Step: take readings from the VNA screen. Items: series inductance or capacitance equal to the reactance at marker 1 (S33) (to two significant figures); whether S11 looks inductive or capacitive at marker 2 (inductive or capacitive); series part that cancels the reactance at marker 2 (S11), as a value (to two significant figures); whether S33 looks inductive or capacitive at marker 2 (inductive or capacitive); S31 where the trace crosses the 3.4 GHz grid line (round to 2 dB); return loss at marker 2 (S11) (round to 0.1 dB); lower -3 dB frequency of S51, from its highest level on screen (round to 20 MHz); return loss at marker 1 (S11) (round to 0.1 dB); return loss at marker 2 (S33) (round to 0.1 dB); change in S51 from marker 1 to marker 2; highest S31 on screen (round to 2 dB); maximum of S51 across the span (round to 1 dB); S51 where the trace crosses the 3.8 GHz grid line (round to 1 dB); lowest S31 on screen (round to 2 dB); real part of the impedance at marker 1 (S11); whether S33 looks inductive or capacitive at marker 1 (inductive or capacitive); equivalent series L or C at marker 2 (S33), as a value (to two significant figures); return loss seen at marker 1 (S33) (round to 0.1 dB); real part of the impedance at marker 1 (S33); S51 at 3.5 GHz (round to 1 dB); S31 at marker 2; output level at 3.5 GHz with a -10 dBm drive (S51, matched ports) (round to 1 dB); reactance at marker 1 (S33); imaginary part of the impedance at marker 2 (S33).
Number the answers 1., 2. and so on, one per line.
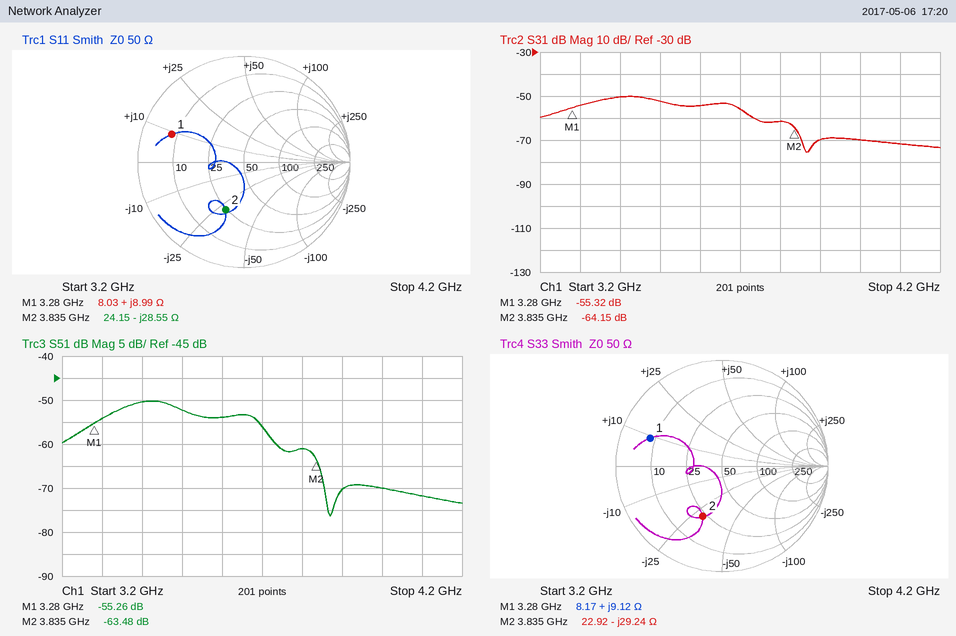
1. 440 pH
2. capacitive
3. 1.2 nH
4. capacitive
5. -50 dB
6. 6.3 dB
7. 3.32 GHz
8. 2.7 dB
9. 5.9 dB
10. -8.22 dB
11. -50 dB
12. -50 dB
13. -61 dB
14. -76 dB
15. 8.03 Ω
16. inductive
17. 1.4 pF
18. 2.8 dB
19. 8.17 Ω
20. -52 dB
21. -64.15 dB
22. -62 dBm
23. +9.12 Ω
24. -29.24 Ω
